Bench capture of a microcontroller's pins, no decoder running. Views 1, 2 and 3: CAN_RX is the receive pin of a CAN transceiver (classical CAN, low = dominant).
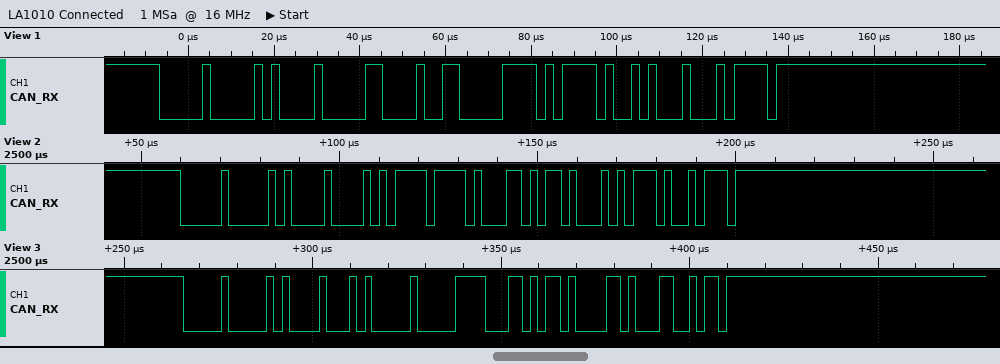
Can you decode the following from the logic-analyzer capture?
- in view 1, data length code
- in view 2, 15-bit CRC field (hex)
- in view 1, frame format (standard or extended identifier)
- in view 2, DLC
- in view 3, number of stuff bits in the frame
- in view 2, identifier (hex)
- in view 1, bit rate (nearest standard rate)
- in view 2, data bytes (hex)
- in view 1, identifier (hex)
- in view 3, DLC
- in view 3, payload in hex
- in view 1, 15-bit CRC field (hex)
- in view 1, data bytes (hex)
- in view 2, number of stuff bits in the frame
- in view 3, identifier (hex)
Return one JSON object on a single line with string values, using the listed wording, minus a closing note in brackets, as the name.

{"in view 1, data length code": "4", "in view 2, 15-bit CRC field": "0x574B", "in view 1, frame format": "standard", "in view 2, DLC": "4", "in view 3, number of stuff bits in the frame": "4", "in view 2, identifier": "0x001", "in view 1, bit rate": "500 kbit/s", "in view 2, data bytes": "2B DE 8D 68", "in view 1, identifier": "0x001", "in view 3, DLC": "4", "in view 3, payload in hex": "50 03 8D 68", "in view 1, 15-bit CRC field": "0x5117", "in view 1, data bytes": "10 98 3A F4", "in view 2, number of stuff bits in the frame": "2", "in view 3, identifier": "0x001"}
